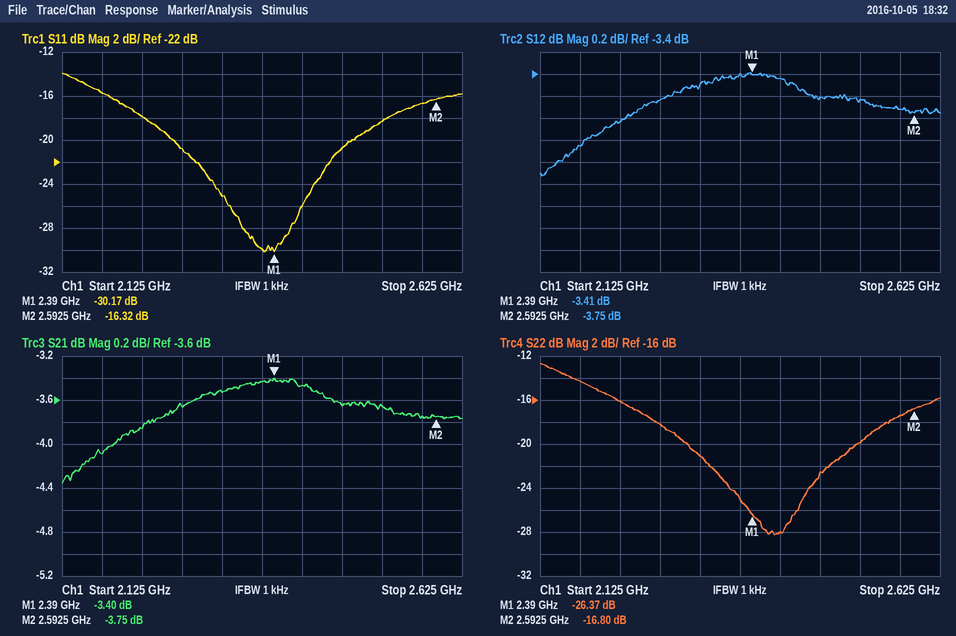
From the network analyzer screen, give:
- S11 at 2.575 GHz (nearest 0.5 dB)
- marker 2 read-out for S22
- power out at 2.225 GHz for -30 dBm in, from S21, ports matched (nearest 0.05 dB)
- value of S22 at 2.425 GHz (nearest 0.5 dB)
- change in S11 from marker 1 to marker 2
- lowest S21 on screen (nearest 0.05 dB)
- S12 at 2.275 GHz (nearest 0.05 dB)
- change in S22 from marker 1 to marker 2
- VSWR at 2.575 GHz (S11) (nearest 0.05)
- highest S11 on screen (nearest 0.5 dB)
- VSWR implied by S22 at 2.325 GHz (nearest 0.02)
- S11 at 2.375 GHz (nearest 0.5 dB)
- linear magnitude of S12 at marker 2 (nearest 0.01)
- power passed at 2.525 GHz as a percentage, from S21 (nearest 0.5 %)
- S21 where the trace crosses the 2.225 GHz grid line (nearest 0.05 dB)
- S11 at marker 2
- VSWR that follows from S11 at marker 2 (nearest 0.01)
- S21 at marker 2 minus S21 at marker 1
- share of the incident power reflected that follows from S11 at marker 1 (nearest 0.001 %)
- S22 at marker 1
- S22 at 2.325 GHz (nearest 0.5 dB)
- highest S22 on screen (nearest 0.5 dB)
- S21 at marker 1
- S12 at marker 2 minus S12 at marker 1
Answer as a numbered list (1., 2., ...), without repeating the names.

1. -16.5 dB
2. -16.80 dB
3. -33.85 dBm
4. -28.0 dB
5. 13.85 dB
6. -4.35 dB
7. -3.65 dB
8. 9.57 dB
9. 1.35
10. -14.0 dB
11. 1.20
12. -30.0 dB
13. 0.65
14. 43.0 %
15. -3.85 dB
16. -16.32 dB
17. 1.36
18. -0.35 dB
19. 0.096 %
20. -26.37 dB
21. -21.0 dB
22. -12.5 dB
23. -3.40 dB
24. -0.34 dB
